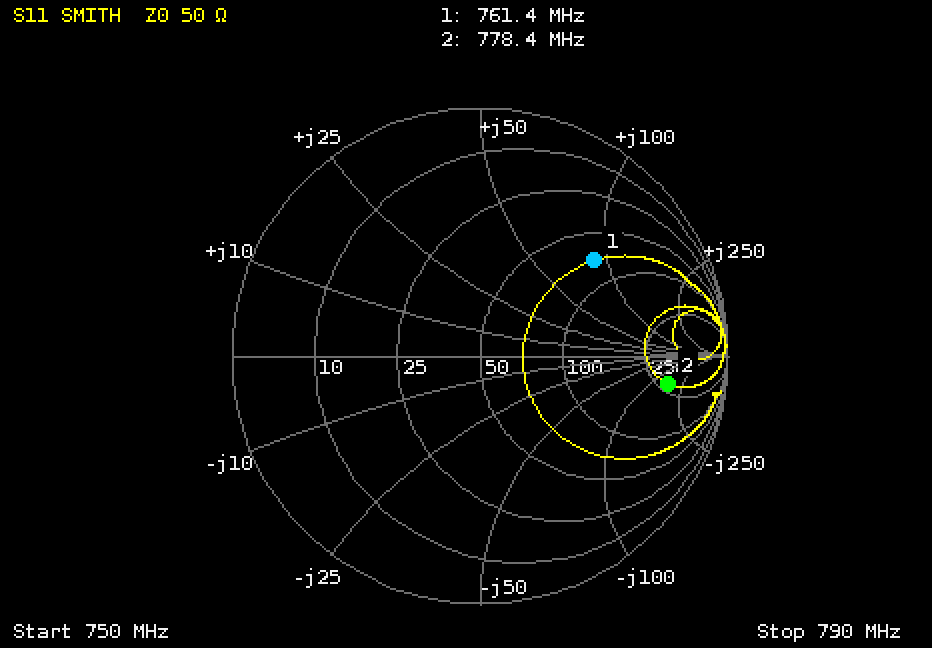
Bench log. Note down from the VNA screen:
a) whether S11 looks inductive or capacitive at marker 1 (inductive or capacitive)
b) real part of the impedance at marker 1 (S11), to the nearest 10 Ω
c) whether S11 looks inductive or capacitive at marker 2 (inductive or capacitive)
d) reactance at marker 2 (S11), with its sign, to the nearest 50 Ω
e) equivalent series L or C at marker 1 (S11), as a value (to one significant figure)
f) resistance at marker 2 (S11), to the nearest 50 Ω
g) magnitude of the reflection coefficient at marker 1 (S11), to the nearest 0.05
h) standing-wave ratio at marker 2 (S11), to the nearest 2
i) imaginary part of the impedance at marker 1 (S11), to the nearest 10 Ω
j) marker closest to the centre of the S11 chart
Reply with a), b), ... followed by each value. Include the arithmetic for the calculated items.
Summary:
a) inductive
b) 70 Ω
c) capacitive
d) -150 Ω
e) L = 90 Ω/(2π × 761.4 MHz) ≈ 18.8 nH, so 20 nH to one significant figure
f) 300 Ω
g) 0.60
h) 8
i) +90 Ω
j) marker 1
